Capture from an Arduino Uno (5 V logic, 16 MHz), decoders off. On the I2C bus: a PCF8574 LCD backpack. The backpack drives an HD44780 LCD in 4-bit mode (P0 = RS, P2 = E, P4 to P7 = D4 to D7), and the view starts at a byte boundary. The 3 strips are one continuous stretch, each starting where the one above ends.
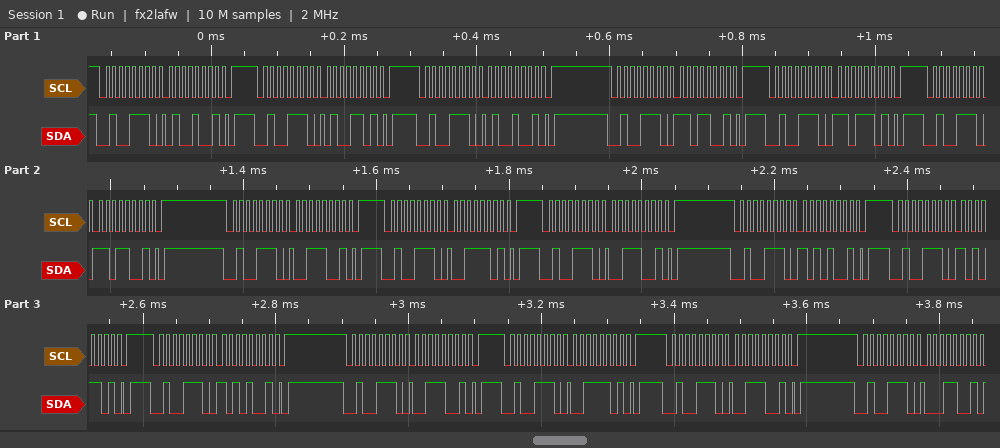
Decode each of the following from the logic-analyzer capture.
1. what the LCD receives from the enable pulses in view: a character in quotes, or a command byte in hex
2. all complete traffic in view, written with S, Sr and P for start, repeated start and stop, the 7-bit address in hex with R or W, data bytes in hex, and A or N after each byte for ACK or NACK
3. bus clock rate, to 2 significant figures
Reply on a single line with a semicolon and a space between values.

'M' ':'; S 27W A 49 A P S 27W A 4D A P S 27W A 49 A P S 27W A D9 A P S 27W A DD A P S 27W A D9 A P S 27W A 39 A P S 27W A 3D A P S 27W A 39 A P S 27W A A9 A P S 27W A AD A P S 27W A A9 A P S 27W A 39 A P S 27W A 3D A P S 27W A 39 A P S 27W A 19 A; 100 kHz
